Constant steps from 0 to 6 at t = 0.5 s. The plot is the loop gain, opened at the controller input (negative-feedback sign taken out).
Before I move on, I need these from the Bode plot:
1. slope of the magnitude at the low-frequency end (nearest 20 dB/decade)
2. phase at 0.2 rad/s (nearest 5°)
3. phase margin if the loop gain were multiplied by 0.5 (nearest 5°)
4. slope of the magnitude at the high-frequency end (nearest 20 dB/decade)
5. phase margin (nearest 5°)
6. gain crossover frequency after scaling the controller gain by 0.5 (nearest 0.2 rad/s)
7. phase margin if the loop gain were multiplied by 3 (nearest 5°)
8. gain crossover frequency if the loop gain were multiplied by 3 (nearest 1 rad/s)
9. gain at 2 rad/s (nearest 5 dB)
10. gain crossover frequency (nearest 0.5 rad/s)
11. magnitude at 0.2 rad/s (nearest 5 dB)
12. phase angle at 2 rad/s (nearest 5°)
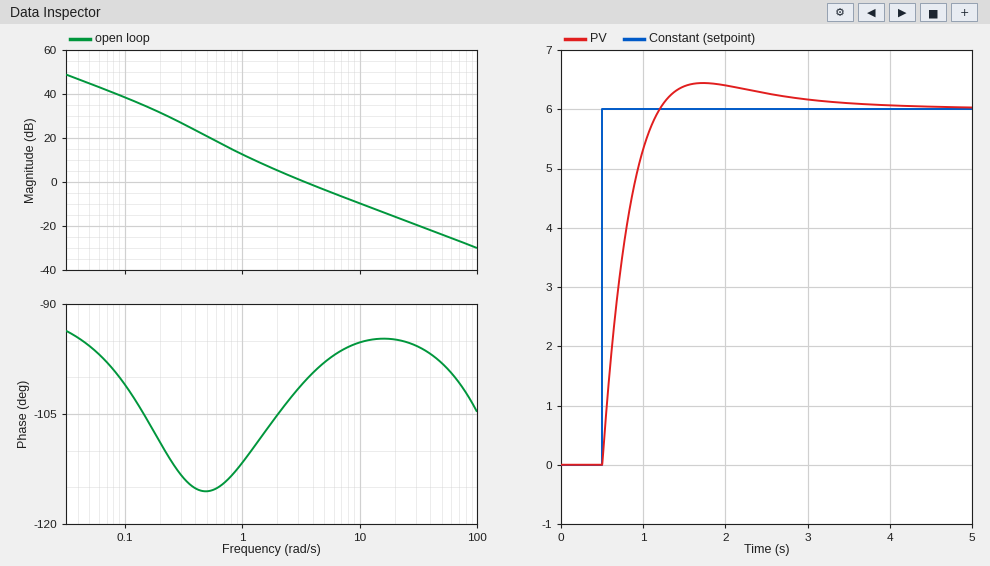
-20 dB/decade
-110°
75°
-20 dB/decade
80°
1.8 rad/s
85°
10 rad/s
5 dB
3.5 rad/s
30 dB
-105°
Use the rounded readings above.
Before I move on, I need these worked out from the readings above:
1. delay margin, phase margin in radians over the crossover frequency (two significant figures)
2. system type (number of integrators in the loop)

0.40 s
1
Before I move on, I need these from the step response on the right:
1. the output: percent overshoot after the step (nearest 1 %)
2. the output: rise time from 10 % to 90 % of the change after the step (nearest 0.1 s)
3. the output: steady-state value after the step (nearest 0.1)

7 %
0.5 s
6.0
